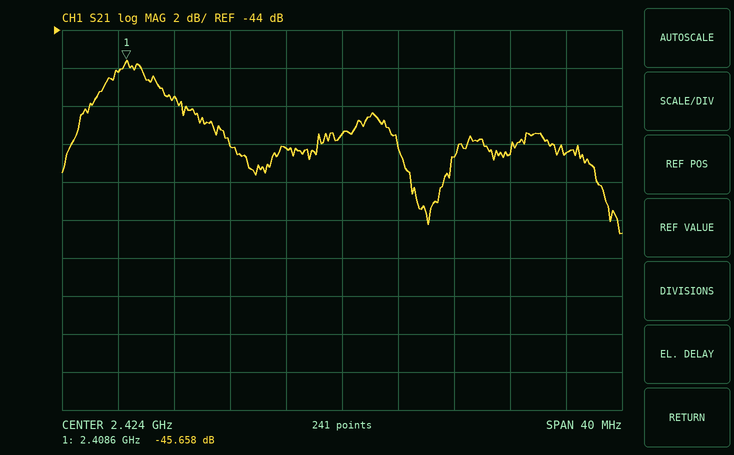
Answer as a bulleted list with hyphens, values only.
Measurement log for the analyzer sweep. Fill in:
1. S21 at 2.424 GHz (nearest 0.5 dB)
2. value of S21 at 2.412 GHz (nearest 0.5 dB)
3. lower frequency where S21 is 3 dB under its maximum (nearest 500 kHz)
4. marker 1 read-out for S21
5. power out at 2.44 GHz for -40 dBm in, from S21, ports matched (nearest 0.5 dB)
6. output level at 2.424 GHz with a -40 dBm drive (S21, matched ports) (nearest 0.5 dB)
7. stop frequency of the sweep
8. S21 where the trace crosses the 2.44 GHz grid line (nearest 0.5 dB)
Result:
- -49.5 dB
- -47.5 dB
- 2.4055 GHz
- -45.658 dB
- -90.5 dBm
- -89.5 dBm
- 2.444 GHz
- -50.5 dB
